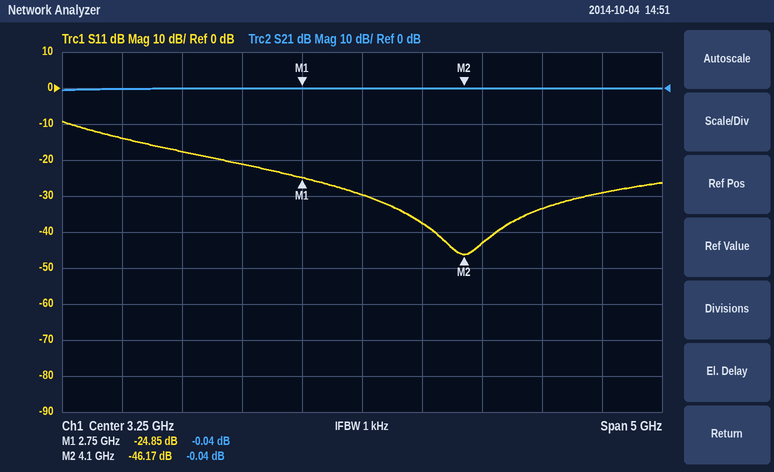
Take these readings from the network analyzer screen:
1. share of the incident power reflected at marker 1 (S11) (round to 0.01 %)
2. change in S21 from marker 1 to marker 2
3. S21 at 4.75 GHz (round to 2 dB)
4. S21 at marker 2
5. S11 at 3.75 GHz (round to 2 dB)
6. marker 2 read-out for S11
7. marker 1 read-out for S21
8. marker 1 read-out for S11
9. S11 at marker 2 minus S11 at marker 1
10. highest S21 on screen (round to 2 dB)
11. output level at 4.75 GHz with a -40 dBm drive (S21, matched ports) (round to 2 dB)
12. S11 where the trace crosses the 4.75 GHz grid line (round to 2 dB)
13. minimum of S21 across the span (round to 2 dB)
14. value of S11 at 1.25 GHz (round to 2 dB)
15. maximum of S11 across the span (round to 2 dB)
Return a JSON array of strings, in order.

["0.33 %", "0.00 dB", "0 dB", "-0.04 dB", "-38 dB", "-46.17 dB", "-0.04 dB", "-24.85 dB", "-21.32 dB", "0 dB", "-40 dBm", "-34 dB", "0 dB", "-14 dB", "-10 dB"]
